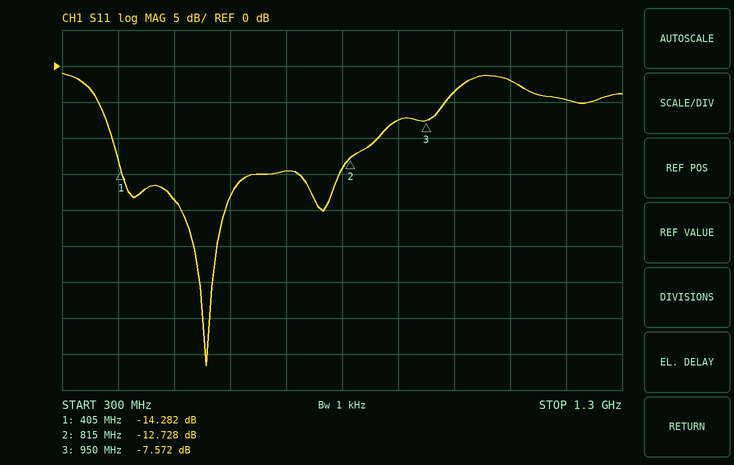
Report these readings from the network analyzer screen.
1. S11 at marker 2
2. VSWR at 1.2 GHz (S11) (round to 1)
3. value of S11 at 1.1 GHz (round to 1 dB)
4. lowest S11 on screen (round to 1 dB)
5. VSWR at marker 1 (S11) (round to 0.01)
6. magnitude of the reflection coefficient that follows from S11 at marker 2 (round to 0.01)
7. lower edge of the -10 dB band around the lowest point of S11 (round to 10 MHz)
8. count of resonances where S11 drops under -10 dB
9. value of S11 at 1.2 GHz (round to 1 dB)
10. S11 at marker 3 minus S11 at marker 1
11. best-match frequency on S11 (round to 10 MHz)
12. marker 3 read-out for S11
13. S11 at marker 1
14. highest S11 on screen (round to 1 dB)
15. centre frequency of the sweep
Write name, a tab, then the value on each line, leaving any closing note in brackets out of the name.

S11 at marker 2	-12.728 dB
VSWR at 1.2 GHz (S11)	4
value of S11 at 1.1 GHz	-2 dB
lowest S11 on screen	-42 dB
VSWR at marker 1 (S11)	1.48
magnitude of the reflection coefficient that follows from S11 at marker 2	0.23
lower edge of the -10 dB band around the lowest point of S11	390 MHz
count of resonances where S11 drops under -10 dB	2
value of S11 at 1.2 GHz	-5 dB
S11 at marker 3 minus S11 at marker 1	6.710 dB
best-match frequency on S11	560 MHz
marker 3 read-out for S11	-7.572 dB
S11 at marker 1	-14.282 dB
highest S11 on screen	-1 dB
centre frequency of the sweep	800 MHz
